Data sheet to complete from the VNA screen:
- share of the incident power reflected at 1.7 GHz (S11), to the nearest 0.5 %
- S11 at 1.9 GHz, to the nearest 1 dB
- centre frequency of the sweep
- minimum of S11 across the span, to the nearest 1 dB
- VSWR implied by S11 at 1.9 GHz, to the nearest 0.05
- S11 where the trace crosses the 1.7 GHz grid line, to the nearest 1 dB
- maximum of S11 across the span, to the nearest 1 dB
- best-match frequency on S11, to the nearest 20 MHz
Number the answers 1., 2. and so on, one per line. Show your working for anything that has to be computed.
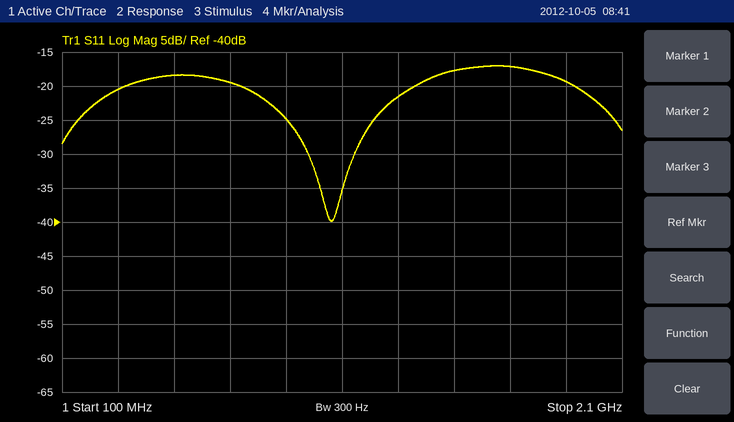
1. 10^(-17/10) ≈ 2.0 %
2. -19 dB
3. 1.1 GHz
4. -40 dB
5. |Γ| = 10^(-19/20) = 0.1122; VSWR = (1 + 0.1122)/(1 − 0.1122) ≈ 1.25
6. -17 dB
7. -17 dB
8. 1.06 GHz
